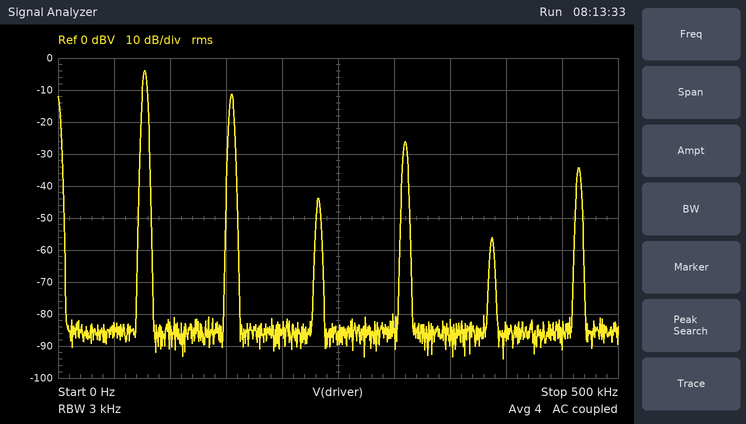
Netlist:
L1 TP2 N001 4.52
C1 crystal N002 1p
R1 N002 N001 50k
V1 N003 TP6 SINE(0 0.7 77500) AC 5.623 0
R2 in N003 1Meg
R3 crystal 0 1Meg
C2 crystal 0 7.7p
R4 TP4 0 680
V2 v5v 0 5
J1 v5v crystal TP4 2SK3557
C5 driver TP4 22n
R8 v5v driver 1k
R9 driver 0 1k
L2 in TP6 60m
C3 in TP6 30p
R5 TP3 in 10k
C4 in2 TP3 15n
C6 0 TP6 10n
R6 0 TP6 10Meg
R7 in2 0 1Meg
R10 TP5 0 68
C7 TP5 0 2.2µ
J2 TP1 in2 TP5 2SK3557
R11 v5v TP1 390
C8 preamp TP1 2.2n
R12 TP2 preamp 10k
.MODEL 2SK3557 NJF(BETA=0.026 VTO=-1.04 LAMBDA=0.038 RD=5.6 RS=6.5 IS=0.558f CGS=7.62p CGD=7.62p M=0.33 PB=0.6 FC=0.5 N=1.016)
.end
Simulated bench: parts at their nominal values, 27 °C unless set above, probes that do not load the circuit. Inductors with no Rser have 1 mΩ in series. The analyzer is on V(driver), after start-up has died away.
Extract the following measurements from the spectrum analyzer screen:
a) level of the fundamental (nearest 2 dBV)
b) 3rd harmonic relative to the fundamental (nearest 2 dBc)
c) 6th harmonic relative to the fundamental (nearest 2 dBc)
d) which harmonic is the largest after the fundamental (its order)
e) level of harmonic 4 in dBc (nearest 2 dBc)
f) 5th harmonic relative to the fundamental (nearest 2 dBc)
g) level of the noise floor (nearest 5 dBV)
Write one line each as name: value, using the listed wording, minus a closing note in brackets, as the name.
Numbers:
level of the fundamental: -4 dBV
3rd harmonic relative to the fundamental: -40 dBc
6th harmonic relative to the fundamental: -30 dBc
which harmonic is the largest after the fundamental: 2
level of harmonic 4 in dBc: -22 dBc
5th harmonic relative to the fundamental: -52 dBc
level of the noise floor: -85 dBV
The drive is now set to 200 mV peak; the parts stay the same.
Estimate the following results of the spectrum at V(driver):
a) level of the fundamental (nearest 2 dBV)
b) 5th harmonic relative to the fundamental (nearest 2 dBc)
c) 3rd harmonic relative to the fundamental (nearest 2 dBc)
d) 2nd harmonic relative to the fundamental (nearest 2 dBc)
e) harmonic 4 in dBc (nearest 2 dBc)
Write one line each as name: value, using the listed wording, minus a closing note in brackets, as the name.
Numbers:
level of the fundamental: -10 dBV
5th harmonic relative to the fundamental: -44 dBc
3rd harmonic relative to the fundamental: -30 dBc
2nd harmonic relative to the fundamental: -22 dBc
harmonic 4 in dBc: -38 dBc
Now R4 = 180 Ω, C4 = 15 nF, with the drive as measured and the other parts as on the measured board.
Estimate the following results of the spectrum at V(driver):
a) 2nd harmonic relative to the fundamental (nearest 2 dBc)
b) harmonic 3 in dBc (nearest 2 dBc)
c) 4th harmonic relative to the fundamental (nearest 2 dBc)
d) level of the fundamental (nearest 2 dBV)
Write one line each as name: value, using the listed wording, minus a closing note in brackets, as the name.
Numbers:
2nd harmonic relative to the fundamental: -10 dBc
harmonic 3 in dBc: -24 dBc
4th harmonic relative to the fundamental: -30 dBc
level of the fundamental: -2 dBV
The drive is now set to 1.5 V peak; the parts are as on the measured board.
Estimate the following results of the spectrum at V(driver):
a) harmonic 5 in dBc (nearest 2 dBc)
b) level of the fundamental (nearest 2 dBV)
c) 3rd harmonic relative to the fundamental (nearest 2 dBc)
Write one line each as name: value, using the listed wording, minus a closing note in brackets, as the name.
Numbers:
harmonic 5 in dBc: -32 dBc
level of the fundamental: -2 dBV
3rd harmonic relative to the fundamental: -26 dBc
